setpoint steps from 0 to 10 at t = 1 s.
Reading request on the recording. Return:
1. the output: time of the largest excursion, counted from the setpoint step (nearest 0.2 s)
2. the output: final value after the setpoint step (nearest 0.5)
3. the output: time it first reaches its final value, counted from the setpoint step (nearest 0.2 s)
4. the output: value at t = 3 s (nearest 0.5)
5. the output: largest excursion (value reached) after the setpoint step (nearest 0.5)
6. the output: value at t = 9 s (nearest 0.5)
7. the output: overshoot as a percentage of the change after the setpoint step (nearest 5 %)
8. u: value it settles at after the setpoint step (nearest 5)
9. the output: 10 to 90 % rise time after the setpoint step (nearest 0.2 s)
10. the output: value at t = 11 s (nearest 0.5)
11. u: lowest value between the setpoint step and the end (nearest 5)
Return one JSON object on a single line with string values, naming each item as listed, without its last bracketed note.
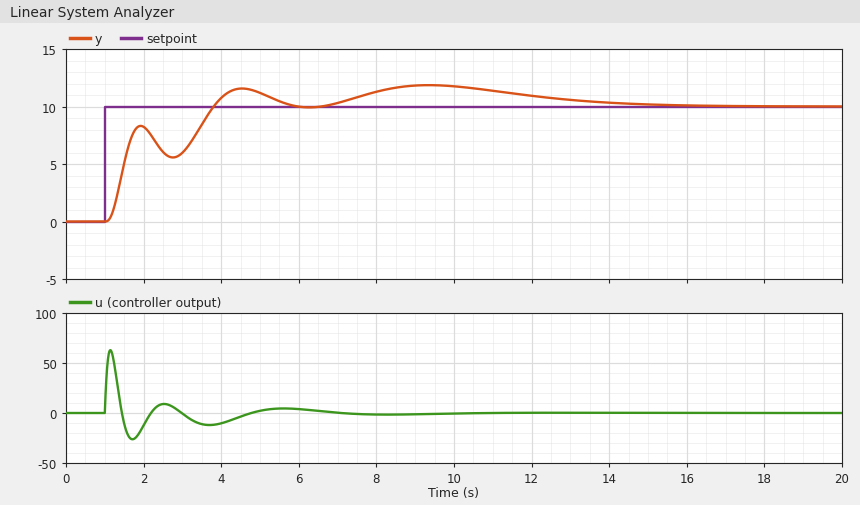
{"the output: time of the largest excursion, counted from the setpoint step": "8.4 s", "the output: final value after the setpoint step": "10.0", "the output: time it first reaches its final value, counted from the setpoint step": "2.8 s", "the output: value at t = 3 s": "6.0", "the output: largest excursion (value reached) after the setpoint step": "12.0", "the output: value at t = 9 s": "12.0", "the output: overshoot as a percentage of the change after the setpoint step": "20 %", "u: value it settles at after the setpoint step": "0", "the output: 10 to 90 % rise time after the setpoint step": "2.4 s", "the output: value at t = 11 s": "11.5", "u: lowest value between the setpoint step and the end": "-25"}
